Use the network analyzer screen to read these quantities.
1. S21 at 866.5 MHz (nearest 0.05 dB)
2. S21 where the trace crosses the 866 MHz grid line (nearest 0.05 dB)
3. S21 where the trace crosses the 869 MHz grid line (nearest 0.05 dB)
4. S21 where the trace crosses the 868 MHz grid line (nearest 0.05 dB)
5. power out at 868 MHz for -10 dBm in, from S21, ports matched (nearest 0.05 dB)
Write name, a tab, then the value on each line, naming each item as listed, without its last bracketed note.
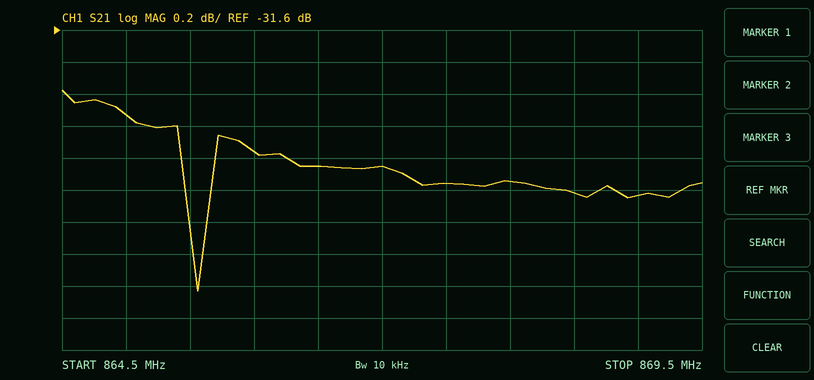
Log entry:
S21 at 866.5 MHz	-32.45 dB
S21 where the trace crosses the 866 MHz grid line	-32.35 dB
S21 where the trace crosses the 869 MHz grid line	-32.65 dB
S21 where the trace crosses the 868 MHz grid line	-32.55 dB
power out at 868 MHz for -10 dBm in, from S21, ports matched	-42.55 dBm
